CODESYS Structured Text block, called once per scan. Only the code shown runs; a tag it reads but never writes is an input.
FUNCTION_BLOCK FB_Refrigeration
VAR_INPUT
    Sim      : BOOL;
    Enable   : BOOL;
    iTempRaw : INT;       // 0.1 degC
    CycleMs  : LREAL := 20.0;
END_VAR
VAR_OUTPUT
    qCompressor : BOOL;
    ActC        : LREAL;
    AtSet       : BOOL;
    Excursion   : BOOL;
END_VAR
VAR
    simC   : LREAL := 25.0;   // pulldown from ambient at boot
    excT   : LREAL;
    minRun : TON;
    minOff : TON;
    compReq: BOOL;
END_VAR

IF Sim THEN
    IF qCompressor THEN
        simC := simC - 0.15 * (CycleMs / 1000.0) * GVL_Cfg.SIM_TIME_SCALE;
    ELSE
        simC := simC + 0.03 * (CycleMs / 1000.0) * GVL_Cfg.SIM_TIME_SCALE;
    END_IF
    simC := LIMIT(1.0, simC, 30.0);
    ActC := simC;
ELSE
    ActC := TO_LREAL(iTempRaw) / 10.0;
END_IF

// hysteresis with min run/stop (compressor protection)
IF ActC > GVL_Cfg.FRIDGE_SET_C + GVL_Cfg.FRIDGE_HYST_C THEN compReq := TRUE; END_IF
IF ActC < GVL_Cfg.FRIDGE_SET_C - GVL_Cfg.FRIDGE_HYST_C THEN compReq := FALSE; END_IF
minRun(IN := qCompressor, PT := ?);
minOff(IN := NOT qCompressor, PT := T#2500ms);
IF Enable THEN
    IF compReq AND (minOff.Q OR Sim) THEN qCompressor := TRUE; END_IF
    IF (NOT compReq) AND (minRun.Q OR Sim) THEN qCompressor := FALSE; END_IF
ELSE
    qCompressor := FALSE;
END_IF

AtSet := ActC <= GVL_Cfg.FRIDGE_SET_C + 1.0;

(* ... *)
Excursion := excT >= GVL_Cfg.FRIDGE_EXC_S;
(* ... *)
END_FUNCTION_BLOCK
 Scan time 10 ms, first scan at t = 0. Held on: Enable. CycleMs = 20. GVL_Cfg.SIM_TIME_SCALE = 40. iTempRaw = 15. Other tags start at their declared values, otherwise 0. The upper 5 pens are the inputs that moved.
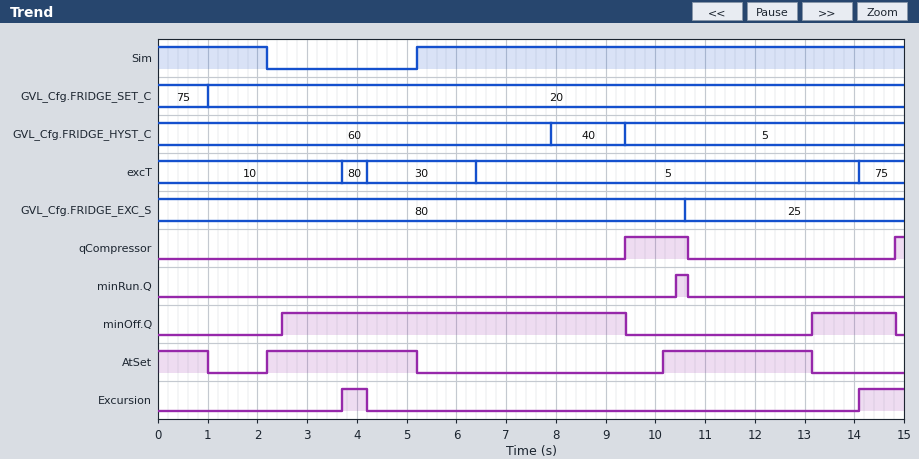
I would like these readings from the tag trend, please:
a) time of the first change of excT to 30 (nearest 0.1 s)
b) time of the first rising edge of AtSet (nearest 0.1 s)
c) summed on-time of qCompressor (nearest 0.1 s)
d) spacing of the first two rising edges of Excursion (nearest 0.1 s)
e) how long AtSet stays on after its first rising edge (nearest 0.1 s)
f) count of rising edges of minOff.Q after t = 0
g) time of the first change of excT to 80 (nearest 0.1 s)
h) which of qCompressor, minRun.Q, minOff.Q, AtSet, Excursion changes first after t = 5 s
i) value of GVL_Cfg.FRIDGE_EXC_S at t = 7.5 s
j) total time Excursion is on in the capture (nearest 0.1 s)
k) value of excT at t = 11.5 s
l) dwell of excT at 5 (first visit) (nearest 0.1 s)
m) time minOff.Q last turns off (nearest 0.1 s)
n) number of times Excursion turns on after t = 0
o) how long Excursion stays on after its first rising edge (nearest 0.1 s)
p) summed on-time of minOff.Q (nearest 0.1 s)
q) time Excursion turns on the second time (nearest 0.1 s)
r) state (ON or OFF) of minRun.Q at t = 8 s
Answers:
4.2 s
2.2 s
1.4 s
10.4 s
3.0 s
2
3.7 s
AtSet
80
1.4 s
5
7.7 s
14.8 s
2
0.5 s
8.6 s
14.1 s
OFF
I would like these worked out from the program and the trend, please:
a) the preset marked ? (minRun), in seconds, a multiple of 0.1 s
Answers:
1.0 s
